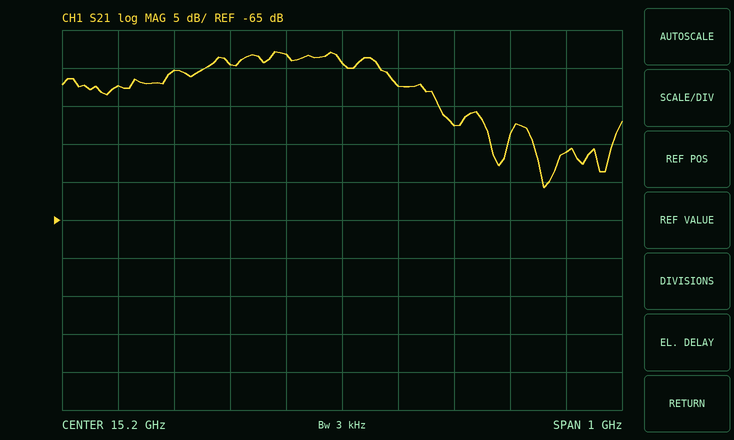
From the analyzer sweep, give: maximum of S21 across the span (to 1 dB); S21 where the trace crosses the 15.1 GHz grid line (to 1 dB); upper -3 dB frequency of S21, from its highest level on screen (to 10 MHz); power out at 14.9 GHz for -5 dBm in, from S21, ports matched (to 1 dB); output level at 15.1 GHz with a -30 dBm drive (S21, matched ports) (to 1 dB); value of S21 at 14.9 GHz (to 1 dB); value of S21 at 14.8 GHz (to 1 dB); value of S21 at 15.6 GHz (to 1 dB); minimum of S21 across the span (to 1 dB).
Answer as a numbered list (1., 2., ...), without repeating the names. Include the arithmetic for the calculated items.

1. -43 dB
2. -43 dB
3. 15.28 GHz
4. -5 dBm + (-45 dB) = -50 dBm
5. -30 dBm + (-43 dB) = -73 dBm
6. -45 dB
7. -47 dB
8. -56 dB
9. -61 dB
